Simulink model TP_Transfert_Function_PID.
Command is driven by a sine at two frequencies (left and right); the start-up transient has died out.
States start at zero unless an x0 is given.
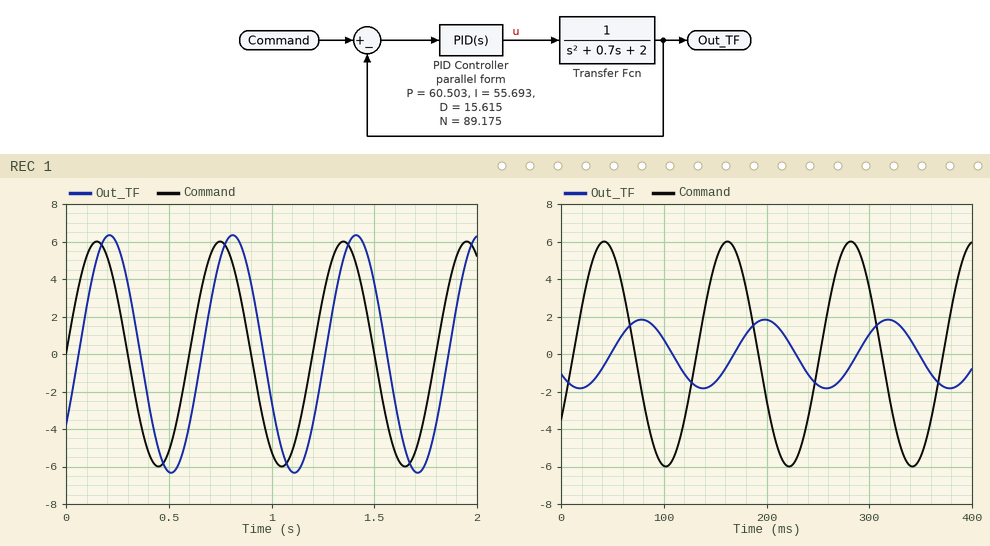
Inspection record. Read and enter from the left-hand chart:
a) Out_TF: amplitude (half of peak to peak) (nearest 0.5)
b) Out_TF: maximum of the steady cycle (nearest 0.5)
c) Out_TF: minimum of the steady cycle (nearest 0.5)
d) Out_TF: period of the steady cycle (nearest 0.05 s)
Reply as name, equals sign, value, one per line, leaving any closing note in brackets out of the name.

Out_TF: amplitude (half of peak to peak) = 6.5
Out_TF: maximum of the steady cycle = 6.5
Out_TF: minimum of the steady cycle = -6.5
Out_TF: period of the steady cycle = 0.60 s
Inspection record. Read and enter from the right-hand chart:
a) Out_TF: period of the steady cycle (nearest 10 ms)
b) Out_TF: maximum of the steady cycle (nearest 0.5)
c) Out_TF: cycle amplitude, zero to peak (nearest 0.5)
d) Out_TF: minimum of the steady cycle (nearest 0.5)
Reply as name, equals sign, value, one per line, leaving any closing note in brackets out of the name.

Out_TF: period of the steady cycle = 120 ms
Out_TF: maximum of the steady cycle = 2.0
Out_TF: cycle amplitude, zero to peak = 2.0
Out_TF: minimum of the steady cycle = -2.0
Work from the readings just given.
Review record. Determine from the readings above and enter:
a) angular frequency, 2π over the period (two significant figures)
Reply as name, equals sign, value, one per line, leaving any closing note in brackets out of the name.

angular frequency, 2π over the period = 0.052 rad/ms
